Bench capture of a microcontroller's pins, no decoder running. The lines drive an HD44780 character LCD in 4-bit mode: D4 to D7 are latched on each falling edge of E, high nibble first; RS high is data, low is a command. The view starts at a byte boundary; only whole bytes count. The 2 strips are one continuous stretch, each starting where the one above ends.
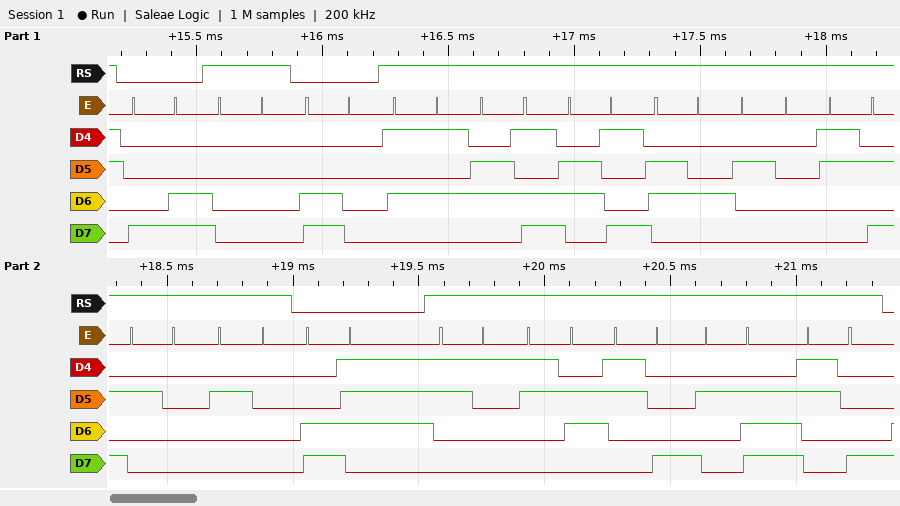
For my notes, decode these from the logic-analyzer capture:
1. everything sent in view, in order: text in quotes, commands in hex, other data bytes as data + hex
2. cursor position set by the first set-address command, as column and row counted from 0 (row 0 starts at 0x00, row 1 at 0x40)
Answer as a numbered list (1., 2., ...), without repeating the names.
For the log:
1. 0x8C data 00 0xC0 "Umid :  " 0xC7 "168.8"
2. column 12, row 0
